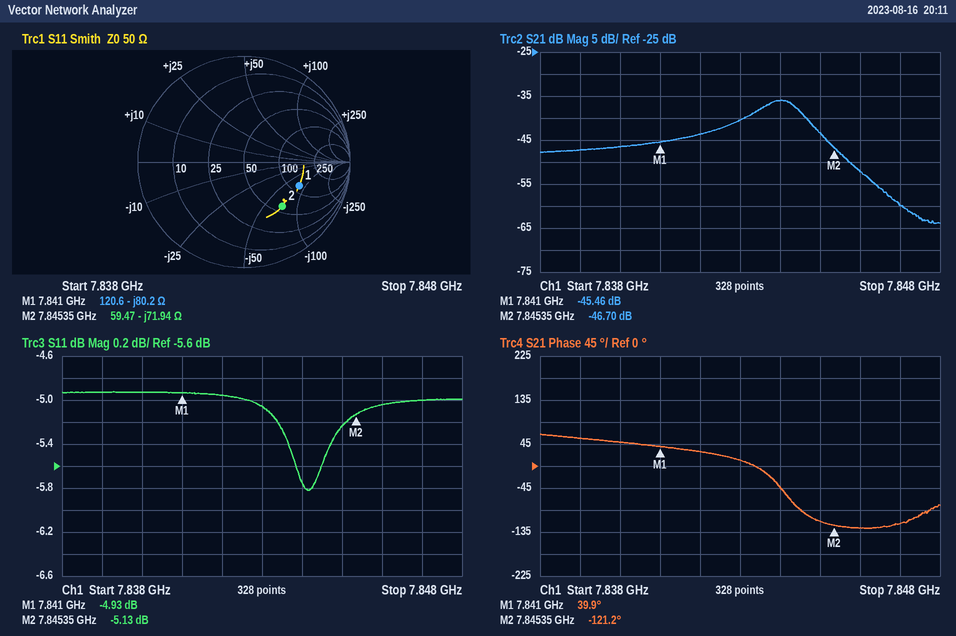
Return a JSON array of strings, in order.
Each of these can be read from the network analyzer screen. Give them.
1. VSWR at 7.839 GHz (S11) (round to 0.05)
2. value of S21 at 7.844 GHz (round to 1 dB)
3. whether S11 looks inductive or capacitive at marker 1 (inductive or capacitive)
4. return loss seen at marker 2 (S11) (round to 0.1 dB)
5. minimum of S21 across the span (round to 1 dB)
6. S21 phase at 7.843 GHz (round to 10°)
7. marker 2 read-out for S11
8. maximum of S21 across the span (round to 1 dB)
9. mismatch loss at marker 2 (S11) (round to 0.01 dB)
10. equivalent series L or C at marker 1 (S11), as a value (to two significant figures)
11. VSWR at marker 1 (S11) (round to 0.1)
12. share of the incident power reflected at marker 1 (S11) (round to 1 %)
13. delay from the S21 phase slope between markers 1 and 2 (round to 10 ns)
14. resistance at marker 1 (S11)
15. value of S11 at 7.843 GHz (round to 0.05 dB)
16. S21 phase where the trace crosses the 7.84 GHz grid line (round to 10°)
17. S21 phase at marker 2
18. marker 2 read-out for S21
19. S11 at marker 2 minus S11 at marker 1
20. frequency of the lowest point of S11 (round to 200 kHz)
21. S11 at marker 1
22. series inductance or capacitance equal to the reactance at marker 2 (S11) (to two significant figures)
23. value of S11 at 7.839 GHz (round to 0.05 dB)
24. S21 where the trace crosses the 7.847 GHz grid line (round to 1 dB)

["3.60", "-36 dB", "capacitive", "5.1 dB", "-64 dB", "10°", "-5.13 dB", "-36 dB", "1.59 dB", "250 fF", "3.6", "32 %", "100 ns", "120.6 Ω", "-5.05 dB", "50°", "-121.2°", "-46.70 dB", "-0.20 dB", "7.8442 GHz", "-4.93 dB", "280 fF", "-4.95 dB", "-60 dB"]
